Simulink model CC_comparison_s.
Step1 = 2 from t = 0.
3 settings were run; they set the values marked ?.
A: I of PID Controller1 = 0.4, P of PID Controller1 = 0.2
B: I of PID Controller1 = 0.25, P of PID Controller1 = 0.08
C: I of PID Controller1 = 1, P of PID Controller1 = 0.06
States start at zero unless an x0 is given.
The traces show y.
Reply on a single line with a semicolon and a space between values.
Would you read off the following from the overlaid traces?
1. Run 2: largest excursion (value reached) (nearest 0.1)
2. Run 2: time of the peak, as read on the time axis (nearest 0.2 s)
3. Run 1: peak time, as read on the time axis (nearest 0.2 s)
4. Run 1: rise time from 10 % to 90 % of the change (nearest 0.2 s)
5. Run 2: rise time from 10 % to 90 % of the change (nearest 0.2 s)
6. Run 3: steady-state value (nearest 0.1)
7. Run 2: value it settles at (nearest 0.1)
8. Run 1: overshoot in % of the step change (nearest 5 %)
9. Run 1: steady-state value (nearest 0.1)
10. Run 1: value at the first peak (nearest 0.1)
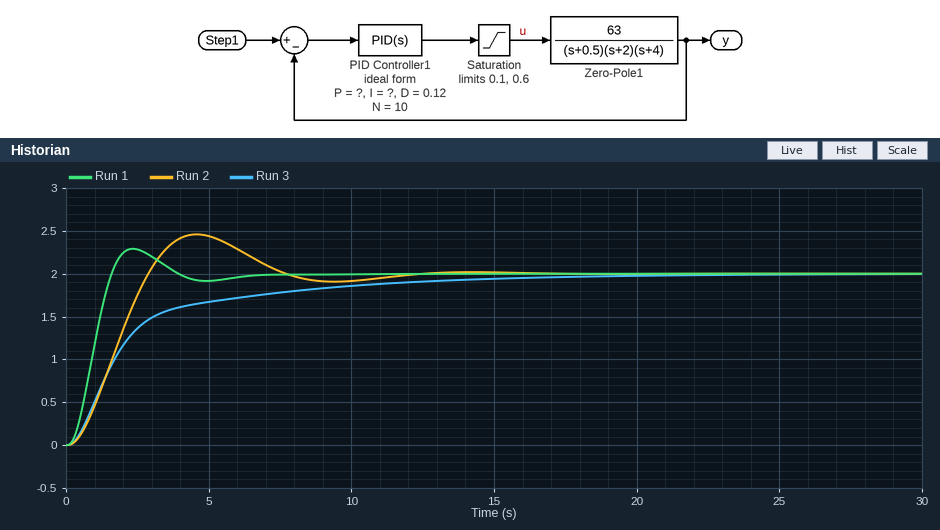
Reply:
2.5; 4.6 s; 2.4 s; 1.0 s; 2.0 s; 2.0; 2.0; 15 %; 2.0; 2.3
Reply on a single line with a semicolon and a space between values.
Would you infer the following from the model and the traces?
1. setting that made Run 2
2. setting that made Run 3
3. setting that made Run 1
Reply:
C; B; A
